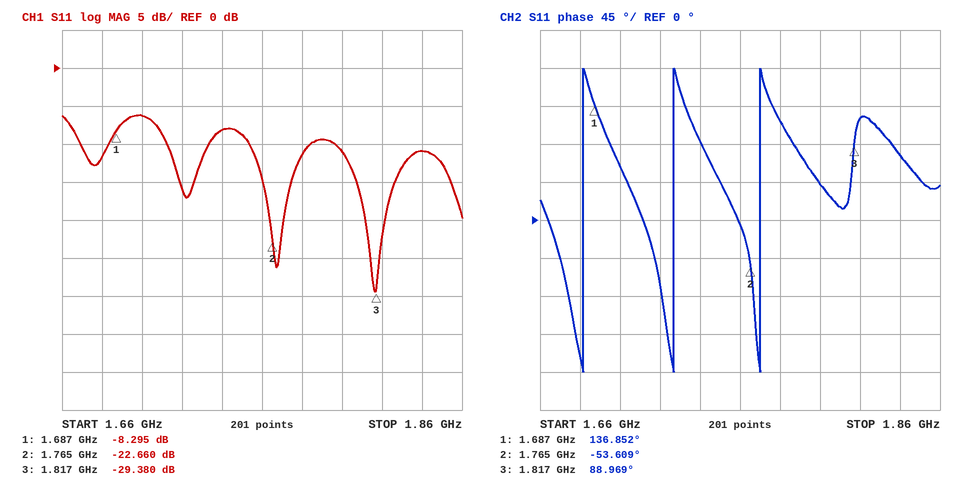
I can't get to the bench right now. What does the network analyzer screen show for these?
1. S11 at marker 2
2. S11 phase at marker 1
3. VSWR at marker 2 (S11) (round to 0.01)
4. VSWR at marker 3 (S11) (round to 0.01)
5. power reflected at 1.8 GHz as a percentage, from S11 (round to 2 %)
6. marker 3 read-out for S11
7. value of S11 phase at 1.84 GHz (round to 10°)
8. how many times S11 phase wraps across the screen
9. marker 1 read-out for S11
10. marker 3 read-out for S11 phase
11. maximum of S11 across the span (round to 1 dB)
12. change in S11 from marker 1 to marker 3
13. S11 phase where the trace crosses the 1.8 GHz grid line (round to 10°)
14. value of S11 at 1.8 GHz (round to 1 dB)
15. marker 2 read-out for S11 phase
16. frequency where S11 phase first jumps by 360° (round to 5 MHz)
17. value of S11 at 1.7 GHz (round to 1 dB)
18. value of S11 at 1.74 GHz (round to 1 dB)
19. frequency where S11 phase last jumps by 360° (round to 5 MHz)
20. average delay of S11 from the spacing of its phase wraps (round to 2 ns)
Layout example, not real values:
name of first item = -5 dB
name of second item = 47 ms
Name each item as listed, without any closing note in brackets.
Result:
S11 at marker 2 = -22.660 dB
S11 phase at marker 1 = 136.852°
VSWR at marker 2 (S11) = 1.16
VSWR at marker 3 (S11) = 1.07
power reflected at 1.8 GHz as a percentage, from S11 = 8 %
marker 3 read-out for S11 = -29.380 dB
value of S11 phase at 1.84 GHz = 80°
how many times S11 phase wraps across the screen = 3
marker 1 read-out for S11 = -8.295 dB
marker 3 read-out for S11 phase = 88.969°
maximum of S11 across the span = -6 dB
change in S11 from marker 1 to marker 3 = -21.085 dB
S11 phase where the trace crosses the 1.8 GHz grid line = 40°
value of S11 at 1.8 GHz = -11 dB
marker 2 read-out for S11 phase = -53.609°
frequency where S11 phase first jumps by 360° = 1.680 GHz
value of S11 at 1.7 GHz = -6 dB
value of S11 at 1.74 GHz = -8 dB
frequency where S11 phase last jumps by 360° = 1.770 GHz
average delay of S11 from the spacing of its phase wraps = 22 ns
